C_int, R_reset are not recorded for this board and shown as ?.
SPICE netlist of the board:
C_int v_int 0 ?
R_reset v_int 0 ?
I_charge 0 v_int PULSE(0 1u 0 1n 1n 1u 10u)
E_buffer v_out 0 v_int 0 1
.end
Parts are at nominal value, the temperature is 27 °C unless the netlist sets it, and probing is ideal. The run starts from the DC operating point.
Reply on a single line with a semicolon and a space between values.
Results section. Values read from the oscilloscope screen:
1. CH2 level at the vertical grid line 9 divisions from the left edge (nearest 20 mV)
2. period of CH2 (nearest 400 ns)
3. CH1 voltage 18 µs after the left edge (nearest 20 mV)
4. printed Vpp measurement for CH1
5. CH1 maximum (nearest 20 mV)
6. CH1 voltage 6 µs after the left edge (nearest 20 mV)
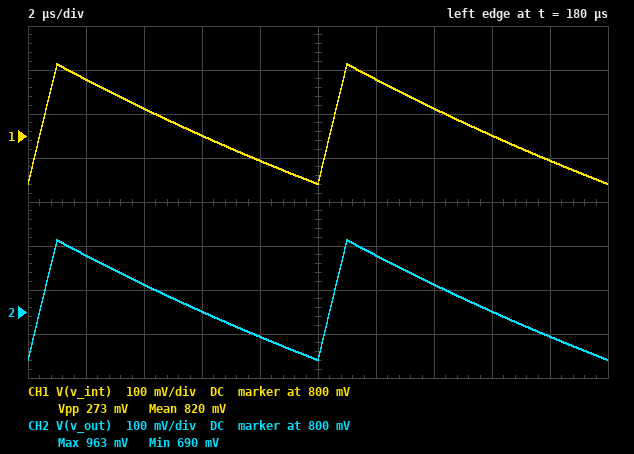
740 mV; 10.0 µs; 740 mV; 273 mV; 960 mV; 800 mV
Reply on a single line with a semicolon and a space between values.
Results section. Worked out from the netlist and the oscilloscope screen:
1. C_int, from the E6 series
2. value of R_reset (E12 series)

3.3 pF; 8.2 MΩ
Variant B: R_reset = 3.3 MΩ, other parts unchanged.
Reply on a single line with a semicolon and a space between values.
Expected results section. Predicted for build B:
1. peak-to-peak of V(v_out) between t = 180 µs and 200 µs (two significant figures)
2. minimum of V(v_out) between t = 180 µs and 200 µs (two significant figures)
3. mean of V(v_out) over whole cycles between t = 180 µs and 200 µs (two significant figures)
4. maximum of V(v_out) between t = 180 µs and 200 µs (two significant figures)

270 mV; 210 mV; 330 mV; 480 mV
